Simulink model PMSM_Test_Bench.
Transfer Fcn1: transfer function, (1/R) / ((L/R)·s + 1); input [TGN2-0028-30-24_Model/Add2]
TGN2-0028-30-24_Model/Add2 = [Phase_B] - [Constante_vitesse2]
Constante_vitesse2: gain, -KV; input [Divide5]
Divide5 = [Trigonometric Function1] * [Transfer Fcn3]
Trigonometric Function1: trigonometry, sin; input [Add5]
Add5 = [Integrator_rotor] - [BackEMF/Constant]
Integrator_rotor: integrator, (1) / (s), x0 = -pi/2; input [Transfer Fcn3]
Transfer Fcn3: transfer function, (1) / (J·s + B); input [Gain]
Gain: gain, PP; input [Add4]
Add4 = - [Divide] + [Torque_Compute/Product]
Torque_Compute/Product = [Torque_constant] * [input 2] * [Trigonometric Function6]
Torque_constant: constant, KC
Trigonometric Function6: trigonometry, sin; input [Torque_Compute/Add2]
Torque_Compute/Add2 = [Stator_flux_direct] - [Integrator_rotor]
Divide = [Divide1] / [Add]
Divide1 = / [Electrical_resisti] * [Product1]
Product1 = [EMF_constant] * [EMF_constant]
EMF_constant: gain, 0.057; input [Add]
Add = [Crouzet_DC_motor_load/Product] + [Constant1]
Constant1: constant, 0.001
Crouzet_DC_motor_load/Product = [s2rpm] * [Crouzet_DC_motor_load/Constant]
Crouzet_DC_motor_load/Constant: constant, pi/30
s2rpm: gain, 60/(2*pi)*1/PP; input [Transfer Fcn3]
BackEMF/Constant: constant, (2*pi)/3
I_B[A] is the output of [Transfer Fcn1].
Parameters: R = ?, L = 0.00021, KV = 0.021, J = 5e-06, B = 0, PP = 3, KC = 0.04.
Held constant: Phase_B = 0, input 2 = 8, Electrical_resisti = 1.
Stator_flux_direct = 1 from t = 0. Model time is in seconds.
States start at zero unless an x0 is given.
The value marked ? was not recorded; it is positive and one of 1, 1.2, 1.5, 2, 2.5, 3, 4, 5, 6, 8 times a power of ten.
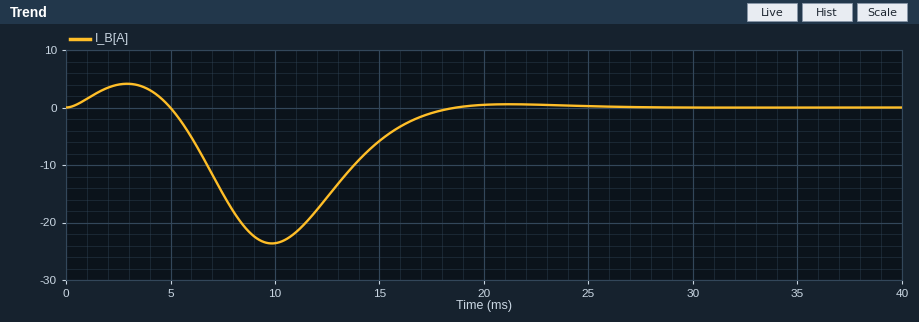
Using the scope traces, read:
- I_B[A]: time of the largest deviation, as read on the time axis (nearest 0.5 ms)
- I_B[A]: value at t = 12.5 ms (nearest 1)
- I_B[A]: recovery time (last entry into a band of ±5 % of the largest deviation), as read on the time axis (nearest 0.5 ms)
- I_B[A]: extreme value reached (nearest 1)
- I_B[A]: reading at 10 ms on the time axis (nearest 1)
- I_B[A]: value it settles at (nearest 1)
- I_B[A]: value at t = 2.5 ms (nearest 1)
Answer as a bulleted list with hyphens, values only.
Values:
- 10.0 ms
- -16
- 17.5 ms
- -24
- -24
- 0
- 4
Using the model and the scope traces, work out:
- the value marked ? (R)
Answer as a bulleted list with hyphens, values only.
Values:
- 0.2
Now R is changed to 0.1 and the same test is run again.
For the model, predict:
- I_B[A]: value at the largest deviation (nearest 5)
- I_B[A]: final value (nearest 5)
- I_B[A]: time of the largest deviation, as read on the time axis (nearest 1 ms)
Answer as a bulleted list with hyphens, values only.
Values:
- -40
- 0
- 11 ms
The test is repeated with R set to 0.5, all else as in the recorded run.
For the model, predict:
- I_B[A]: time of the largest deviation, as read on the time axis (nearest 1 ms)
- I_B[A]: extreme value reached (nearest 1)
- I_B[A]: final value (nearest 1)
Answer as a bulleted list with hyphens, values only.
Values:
- 9 ms
- -10
- 0
